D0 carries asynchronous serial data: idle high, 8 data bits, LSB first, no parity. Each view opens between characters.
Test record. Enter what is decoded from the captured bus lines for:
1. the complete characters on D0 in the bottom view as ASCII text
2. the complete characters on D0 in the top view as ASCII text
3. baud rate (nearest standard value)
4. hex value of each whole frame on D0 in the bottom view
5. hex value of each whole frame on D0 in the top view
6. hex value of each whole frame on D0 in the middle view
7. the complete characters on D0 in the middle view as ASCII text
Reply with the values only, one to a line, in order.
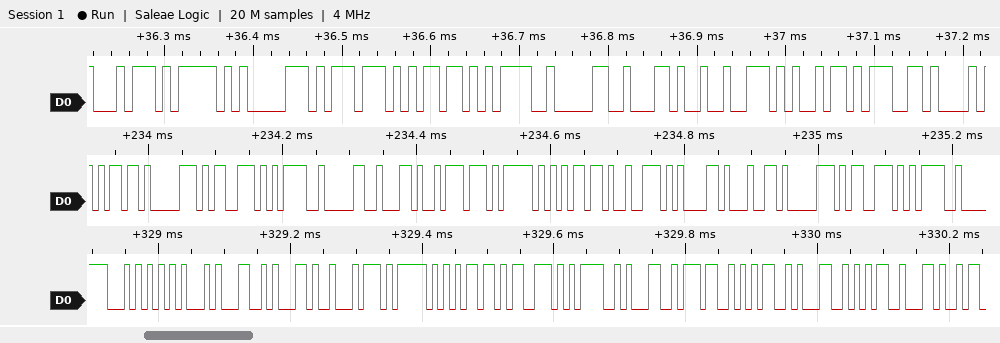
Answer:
"TEL,t_ms=17515,"
"t_pwm=0,rig"
115200 baud
54, 45, 4C, 2C, 74, 5F, 6D, 73, 3D, 31, 37, 35, 31, 35, 2C
74, 5F, 70, 77, 6D, 3D, 30, 2C, 72, 69, 67
6D, 70, 73, 3D, 30, 2C, 77, 5F, 6D, 72, 61, 64, 70, 73, 3D
"mps=0,w_mradps="
